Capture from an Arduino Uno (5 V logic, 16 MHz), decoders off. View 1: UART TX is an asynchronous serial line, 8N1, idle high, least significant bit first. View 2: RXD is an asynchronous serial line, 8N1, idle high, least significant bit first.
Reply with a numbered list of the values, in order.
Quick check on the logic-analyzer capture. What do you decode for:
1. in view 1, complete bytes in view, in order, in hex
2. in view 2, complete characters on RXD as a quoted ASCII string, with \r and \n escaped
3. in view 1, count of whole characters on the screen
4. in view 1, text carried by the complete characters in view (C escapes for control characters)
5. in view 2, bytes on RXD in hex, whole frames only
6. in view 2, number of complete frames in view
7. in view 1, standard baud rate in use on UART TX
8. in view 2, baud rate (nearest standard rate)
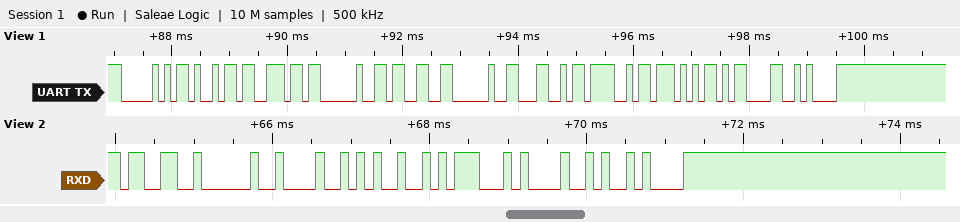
1. 50 69 6E 20 33 20 4C 4F 57 0D 0A
2. "3 HIGH\n"
3. 11
4. "Pin 3 LOW\r\n"
5. 33 20 48 49 47 48 0A
6. 7
7. 9600 baud
8. 9600 baud
